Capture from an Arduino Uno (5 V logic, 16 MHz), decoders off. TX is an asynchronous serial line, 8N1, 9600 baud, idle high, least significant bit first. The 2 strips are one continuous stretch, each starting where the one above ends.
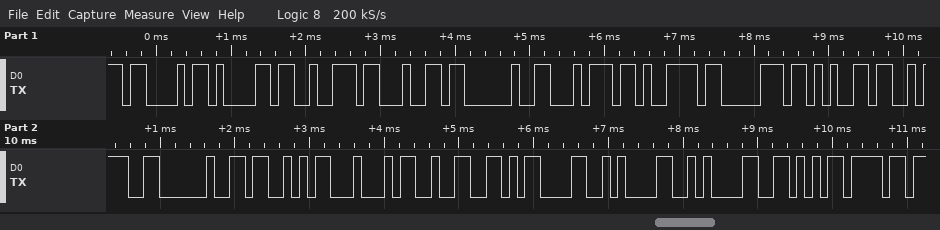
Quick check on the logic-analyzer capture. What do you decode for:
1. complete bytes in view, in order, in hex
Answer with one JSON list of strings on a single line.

["0x43 0x61 0x72 0x64 0x20 0x74 0x79 0x70 0x65 0x3A 0x20 0x53 0x44 0x32 0x0D 0x0A 0x0A 0x56 0x6F"]
